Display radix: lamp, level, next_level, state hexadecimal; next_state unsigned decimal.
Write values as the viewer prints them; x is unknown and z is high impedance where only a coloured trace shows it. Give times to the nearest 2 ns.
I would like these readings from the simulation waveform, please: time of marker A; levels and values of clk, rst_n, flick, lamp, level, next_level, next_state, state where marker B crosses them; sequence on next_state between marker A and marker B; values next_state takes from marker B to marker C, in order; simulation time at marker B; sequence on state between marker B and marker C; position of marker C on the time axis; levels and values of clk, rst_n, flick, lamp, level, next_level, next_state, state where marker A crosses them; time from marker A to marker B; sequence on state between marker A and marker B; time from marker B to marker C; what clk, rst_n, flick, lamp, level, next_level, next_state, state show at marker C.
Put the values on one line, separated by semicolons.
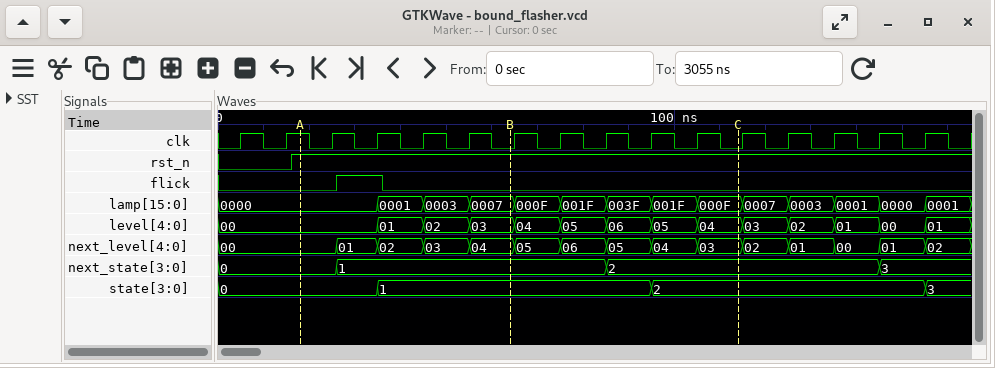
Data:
18 ns; clk=0, rst_n=1, flick=0, lamp=0007, level=03, next_level=04, next_state=1, state=1; 0, 1; 1, 2; 64 ns; 1, 2; 114 ns; clk=1, rst_n=1, flick=0, lamp=0000, level=00, next_level=00, next_state=0, state=0; 46 ns; 0, 1; 50 ns; clk=0, rst_n=1, flick=0, lamp=000F, level=04, next_level=03, next_state=2, state=2
